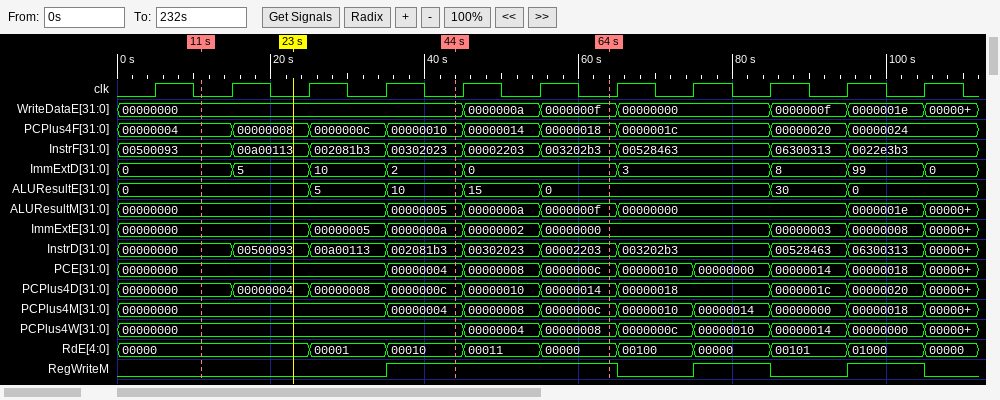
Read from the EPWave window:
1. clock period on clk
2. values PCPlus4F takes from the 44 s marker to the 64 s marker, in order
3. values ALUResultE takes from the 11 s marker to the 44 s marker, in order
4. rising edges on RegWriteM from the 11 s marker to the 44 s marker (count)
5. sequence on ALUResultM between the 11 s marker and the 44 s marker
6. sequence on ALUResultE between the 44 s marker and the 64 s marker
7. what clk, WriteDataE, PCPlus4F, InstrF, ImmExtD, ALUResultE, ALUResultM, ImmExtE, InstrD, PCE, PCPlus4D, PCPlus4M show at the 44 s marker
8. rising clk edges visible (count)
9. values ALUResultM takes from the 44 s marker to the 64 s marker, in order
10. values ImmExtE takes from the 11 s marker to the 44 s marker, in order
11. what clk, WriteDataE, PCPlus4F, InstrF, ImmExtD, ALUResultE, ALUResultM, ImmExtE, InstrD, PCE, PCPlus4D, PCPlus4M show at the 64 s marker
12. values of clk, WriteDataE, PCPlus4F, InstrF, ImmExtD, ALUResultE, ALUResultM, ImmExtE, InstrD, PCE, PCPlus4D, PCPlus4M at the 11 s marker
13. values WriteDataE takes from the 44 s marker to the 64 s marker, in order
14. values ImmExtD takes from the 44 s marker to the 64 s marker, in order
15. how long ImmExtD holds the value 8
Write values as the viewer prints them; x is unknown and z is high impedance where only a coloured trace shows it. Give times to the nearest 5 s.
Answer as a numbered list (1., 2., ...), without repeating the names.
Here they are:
1. 10 s
2. 00000010, 00000014, 00000018
3. 0, 5, 10
4. 1
5. 00000000, 00000005
6. 10, 15, 0
7. clk=0, WriteDataE=00000000, PCPlus4F=00000010, InstrF=00302023, ImmExtD=2, ALUResultE=10, ALUResultM=00000005, ImmExtE=0000000a, InstrD=002081b3, PCE=00000004, PCPlus4D=0000000c, PCPlus4M=00000004
8. 11
9. 00000005, 0000000a, 0000000f
10. 00000000, 00000005, 0000000a
11. clk=0, WriteDataE=0000000f, PCPlus4F=00000018, InstrF=003202b3, ImmExtD=0, ALUResultE=0, ALUResultM=0000000f, ImmExtE=00000000, InstrD=00002203, PCE=0000000c, PCPlus4D=00000014, PCPlus4M=0000000c
12. clk=0, WriteDataE=00000000, PCPlus4F=00000004, InstrF=00500093, ImmExtD=0, ALUResultE=0, ALUResultM=00000000, ImmExtE=00000000, InstrD=00000000, PCE=00000000, PCPlus4D=00000000, PCPlus4M=00000000
13. 00000000, 0000000a, 0000000f
14. 2, 0
15. 10 s
